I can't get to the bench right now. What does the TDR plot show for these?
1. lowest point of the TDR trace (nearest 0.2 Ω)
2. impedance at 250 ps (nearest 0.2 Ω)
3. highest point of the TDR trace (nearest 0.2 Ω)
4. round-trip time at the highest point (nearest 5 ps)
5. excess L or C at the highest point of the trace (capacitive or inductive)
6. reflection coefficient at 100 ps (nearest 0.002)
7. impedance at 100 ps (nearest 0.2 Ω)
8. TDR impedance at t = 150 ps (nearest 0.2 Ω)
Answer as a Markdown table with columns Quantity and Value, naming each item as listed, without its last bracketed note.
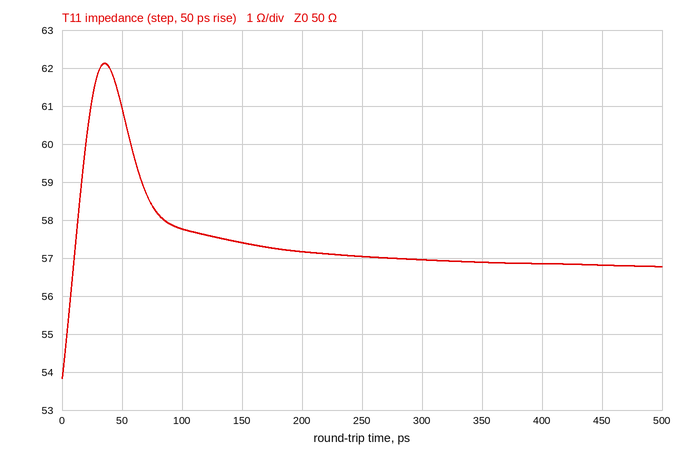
| Quantity | Value |
|---|---|
| lowest point of the TDR trace | 53.8 Ω |
| impedance at 250 ps | 57.0 Ω |
| highest point of the TDR trace | 62.2 Ω |
| round-trip time at the highest point | 35 ps |
| excess L or C at the highest point of the trace | inductive |
| reflection coefficient at 100 ps | +0.072 |
| impedance at 100 ps | 57.8 Ω |
| TDR impedance at t = 150 ps | 57.4 Ω |
